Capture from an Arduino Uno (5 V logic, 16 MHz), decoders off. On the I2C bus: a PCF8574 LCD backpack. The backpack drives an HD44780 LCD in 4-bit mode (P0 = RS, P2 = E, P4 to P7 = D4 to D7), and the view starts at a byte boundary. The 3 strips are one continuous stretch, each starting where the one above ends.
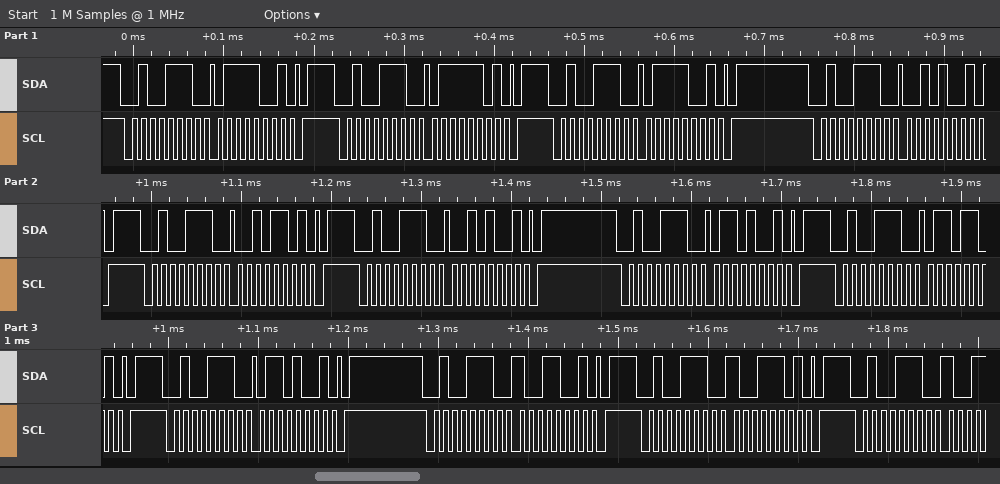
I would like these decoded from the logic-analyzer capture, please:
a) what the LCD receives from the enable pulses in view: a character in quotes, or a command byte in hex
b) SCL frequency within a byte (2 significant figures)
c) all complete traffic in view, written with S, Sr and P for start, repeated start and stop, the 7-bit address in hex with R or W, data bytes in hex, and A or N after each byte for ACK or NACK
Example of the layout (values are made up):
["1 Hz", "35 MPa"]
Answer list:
["'r'", "100 kHz", "S 27W A 79 A P S 27W A 7D A P S 27W A 79 A P S 27W A 29 A P S 27W A 2D A P S 27W A 29 A P S 27W A 69 A P S 27W A 6D A P S 27W A 69 A P S 27W A 99 A P S 27W A 9D A P S 27W A"]
